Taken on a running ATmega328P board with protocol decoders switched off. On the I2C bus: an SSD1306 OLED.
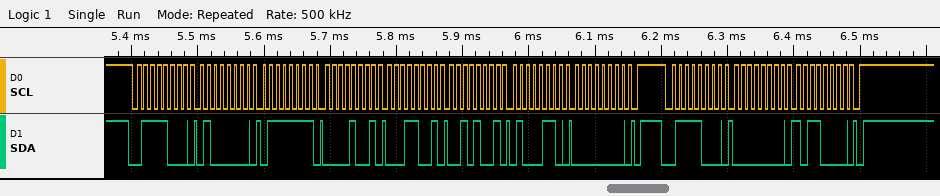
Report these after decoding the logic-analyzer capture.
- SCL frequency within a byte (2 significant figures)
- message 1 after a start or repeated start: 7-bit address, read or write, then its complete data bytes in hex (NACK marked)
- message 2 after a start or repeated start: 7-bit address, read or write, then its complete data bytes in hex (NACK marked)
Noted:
100 kHz
0x3C write: 40 7F 09 19 29 46 00
0x3C write: 00 B0
